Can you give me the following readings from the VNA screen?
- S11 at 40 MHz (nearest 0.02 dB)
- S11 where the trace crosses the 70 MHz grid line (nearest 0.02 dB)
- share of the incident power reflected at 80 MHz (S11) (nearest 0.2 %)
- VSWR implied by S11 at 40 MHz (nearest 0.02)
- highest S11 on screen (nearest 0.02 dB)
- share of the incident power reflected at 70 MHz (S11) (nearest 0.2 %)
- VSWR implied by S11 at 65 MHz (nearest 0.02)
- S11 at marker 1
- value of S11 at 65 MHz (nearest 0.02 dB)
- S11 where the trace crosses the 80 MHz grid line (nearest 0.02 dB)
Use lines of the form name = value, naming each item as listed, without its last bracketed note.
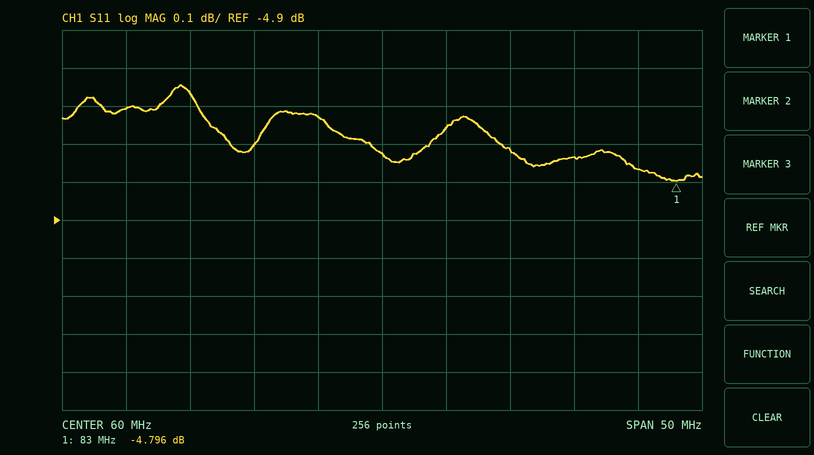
S11 at 40 MHz = -4.60 dB
S11 where the trace crosses the 70 MHz grid line = -4.72 dB
share of the incident power reflected at 80 MHz (S11) = 33.4 %
VSWR implied by S11 at 40 MHz = 3.86
highest S11 on screen = -4.54 dB
share of the incident power reflected at 70 MHz (S11) = 33.8 %
VSWR implied by S11 at 65 MHz = 3.82
S11 at marker 1 = -4.796 dB
value of S11 at 65 MHz = -4.66 dB
S11 where the trace crosses the 80 MHz grid line = -4.76 dB
